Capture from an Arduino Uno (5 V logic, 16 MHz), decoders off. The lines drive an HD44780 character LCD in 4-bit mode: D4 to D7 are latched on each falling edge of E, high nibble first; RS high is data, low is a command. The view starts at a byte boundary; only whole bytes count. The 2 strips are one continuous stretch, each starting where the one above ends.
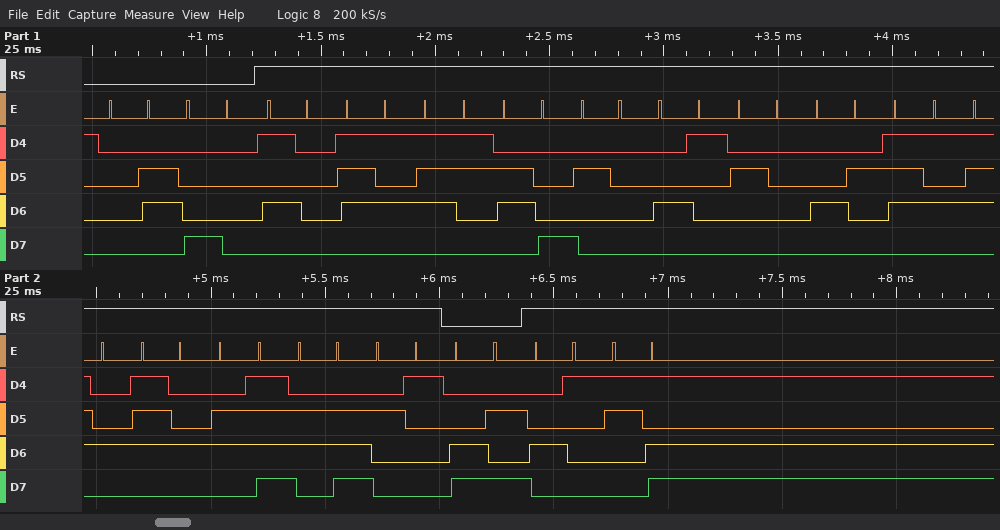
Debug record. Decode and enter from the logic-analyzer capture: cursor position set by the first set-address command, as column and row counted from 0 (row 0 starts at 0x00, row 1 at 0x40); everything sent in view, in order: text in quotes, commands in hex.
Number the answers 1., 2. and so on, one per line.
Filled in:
1. column 0, row 0
2. 0x06 0x80 "Push A Button!" 0xCA "A="
